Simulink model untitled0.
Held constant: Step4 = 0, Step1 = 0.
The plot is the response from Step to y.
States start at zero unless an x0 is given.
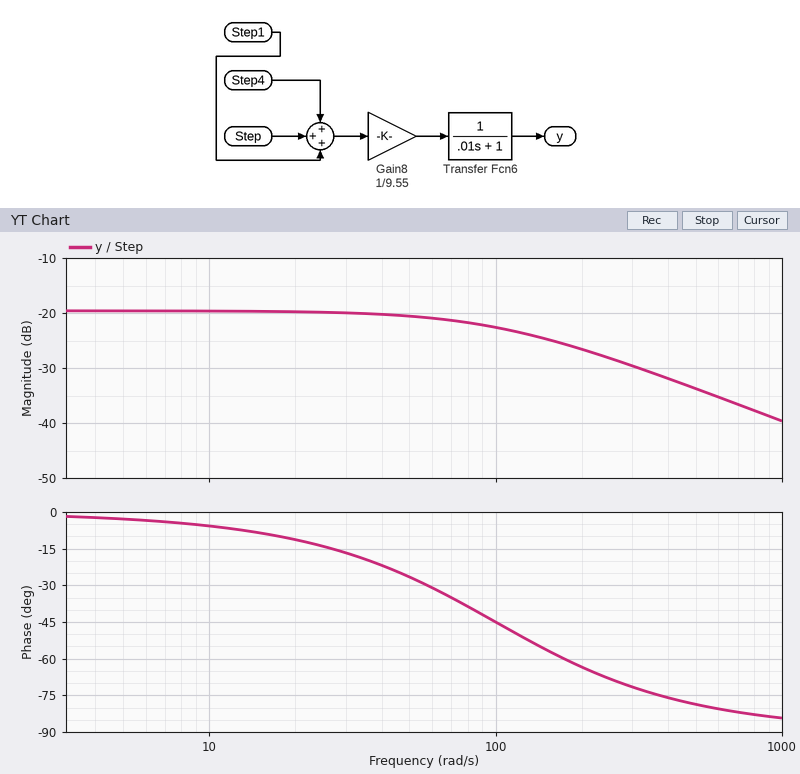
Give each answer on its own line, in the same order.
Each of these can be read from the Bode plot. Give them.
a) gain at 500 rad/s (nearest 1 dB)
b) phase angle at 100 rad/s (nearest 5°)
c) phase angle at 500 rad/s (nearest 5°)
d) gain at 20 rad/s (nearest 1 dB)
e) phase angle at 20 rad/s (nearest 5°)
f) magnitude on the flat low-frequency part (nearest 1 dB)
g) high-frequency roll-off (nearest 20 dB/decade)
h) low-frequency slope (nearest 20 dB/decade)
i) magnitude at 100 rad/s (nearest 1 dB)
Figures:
-34 dB
-45°
-80°
-20 dB
-10°
-20 dB
-20 dB/decade
0 dB/decade
-23 dB
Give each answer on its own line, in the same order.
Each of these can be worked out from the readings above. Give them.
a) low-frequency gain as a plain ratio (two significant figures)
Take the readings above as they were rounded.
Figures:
0.10
